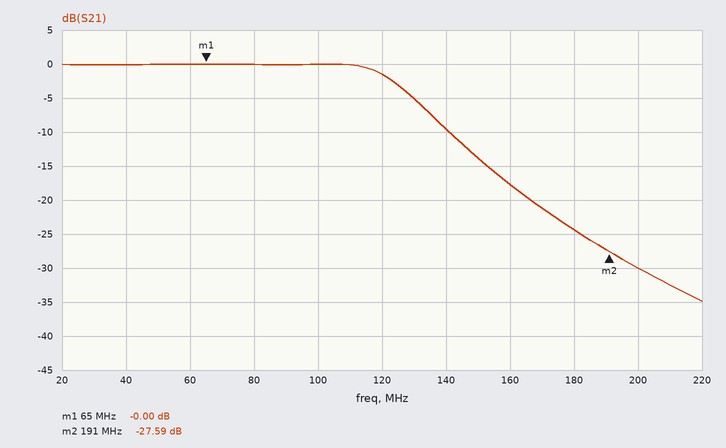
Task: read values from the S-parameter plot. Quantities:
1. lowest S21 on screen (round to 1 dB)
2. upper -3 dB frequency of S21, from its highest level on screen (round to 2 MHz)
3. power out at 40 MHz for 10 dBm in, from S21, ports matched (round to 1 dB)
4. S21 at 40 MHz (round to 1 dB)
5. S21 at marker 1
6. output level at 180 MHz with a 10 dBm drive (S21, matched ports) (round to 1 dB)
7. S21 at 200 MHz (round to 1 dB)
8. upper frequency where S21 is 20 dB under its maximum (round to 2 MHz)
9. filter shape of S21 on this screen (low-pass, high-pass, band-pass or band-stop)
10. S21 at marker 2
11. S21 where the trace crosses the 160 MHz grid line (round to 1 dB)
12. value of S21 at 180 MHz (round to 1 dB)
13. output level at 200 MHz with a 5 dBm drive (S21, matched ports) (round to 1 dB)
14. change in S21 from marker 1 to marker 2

-35 dB
124 MHz
10 dBm
0 dB
-0.00 dB
-14 dBm
-30 dB
166 MHz
low-pass
-27.59 dB
-18 dB
-24 dB
-25 dBm
-27.59 dB
